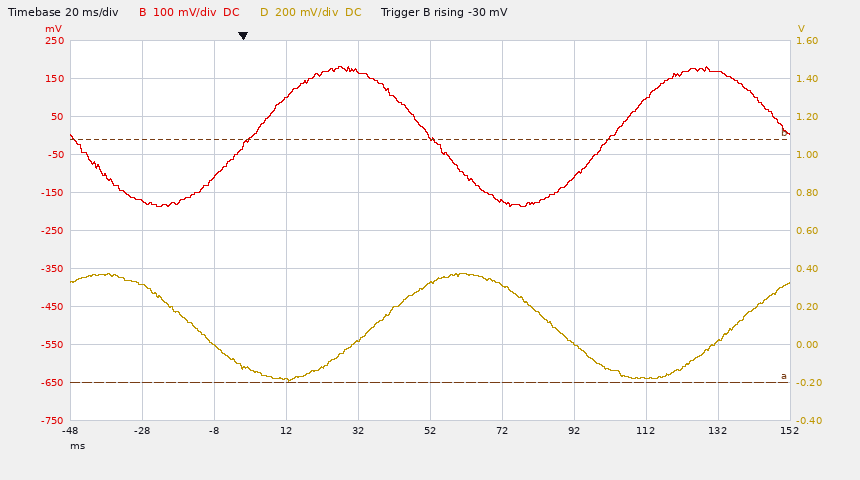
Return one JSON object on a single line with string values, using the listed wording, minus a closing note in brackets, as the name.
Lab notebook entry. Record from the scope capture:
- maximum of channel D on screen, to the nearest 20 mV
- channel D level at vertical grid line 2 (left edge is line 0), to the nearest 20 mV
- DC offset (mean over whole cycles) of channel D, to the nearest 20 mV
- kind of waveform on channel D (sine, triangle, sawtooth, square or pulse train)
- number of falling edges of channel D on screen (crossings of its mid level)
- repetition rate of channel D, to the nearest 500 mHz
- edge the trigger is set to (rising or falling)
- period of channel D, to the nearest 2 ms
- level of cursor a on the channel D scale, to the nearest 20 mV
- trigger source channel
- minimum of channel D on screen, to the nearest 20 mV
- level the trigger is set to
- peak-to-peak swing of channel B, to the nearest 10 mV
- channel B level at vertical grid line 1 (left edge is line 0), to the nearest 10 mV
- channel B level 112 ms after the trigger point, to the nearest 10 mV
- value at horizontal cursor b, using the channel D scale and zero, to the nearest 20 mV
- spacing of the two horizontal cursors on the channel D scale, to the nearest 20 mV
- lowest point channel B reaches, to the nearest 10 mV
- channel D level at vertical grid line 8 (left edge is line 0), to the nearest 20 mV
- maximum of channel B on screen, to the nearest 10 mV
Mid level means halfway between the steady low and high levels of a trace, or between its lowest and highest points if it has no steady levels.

{"maximum of channel D on screen, to the nearest 20 mV": "380 mV", "channel D level at vertical grid line 2 (left edge is line 0), to the nearest 20 mV": "0 mV", "DC offset (mean over whole cycles) of channel D, to the nearest 20 mV": "100 mV", "kind of waveform on channel D": "sine", "number of falling edges of channel D on screen": "2", "repetition rate of channel D, to the nearest 500 mHz": "10.0 Hz", "edge the trigger is set to": "rising", "period of channel D, to the nearest 2 ms": "100 ms", "level of cursor a on the channel D scale, to the nearest 20 mV": "-200 mV", "trigger source channel": "channel B", "minimum of channel D on screen, to the nearest 20 mV": "-200 mV", "level the trigger is set to": "-30 mV", "peak-to-peak swing of channel B, to the nearest 10 mV": "370 mV", "channel B level at vertical grid line 1 (left edge is line 0), to the nearest 10 mV": "-170 mV", "channel B level 112 ms after the trigger point, to the nearest 10 mV": "100 mV", "value at horizontal cursor b, using the channel D scale and zero, to the nearest 20 mV": "1.08 V", "spacing of the two horizontal cursors on the channel D scale, to the nearest 20 mV": "1.28 V", "lowest point channel B reaches, to the nearest 10 mV": "-190 mV", "channel D level at vertical grid line 8 (left edge is line 0), to the nearest 20 mV": "-180 mV", "maximum of channel B on screen, to the nearest 10 mV": "180 mV"}
